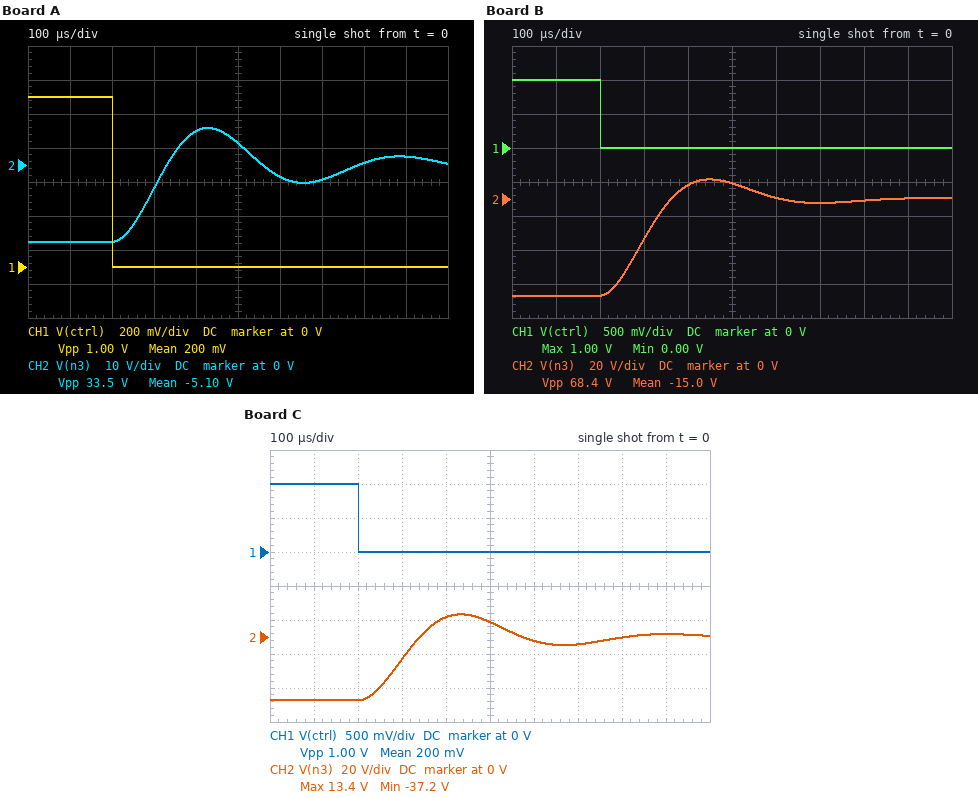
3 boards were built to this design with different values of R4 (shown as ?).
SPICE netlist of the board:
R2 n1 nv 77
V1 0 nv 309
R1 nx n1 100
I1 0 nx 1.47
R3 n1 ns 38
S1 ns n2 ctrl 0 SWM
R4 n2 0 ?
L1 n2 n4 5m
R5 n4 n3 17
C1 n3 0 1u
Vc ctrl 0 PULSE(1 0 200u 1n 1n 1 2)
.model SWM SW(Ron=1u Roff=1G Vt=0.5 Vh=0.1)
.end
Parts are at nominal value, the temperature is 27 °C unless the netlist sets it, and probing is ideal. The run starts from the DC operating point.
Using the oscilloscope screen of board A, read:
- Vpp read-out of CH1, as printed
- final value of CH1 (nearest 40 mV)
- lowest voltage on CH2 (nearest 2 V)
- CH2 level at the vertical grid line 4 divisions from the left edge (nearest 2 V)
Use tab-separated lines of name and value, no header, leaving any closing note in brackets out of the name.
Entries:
Vpp read-out of CH1, as printed	1.00 V
final value of CH1	0 V
lowest voltage on CH2	-22 V
CH2 level at the vertical grid line 4 divisions from the left edge	10 V
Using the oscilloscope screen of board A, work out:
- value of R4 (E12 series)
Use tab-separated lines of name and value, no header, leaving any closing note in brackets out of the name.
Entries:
value of R4	15 Ω
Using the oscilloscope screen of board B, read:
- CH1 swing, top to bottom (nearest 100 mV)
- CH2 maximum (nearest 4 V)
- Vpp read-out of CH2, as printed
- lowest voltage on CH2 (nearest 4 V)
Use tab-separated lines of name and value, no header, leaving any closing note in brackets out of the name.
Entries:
CH1 swing, top to bottom	1.0 V
CH2 maximum	12 V
Vpp read-out of CH2, as printed	68.4 V
lowest voltage on CH2	-56 V
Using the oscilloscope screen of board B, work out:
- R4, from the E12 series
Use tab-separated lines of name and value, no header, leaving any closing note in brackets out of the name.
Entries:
R4, from the E12 series	47 Ω
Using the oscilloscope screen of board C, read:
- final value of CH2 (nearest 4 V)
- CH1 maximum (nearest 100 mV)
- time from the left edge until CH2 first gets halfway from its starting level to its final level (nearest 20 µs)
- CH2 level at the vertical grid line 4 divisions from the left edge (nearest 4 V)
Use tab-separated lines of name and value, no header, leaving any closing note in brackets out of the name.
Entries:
final value of CH2	0 V
CH1 maximum	1.0 V
time from the left edge until CH2 first gets halfway from its starting level to its final level	280 µs
CH2 level at the vertical grid line 4 divisions from the left edge	12 V
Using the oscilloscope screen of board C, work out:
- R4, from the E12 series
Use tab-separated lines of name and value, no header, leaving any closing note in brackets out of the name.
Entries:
R4, from the E12 series	27 Ω
